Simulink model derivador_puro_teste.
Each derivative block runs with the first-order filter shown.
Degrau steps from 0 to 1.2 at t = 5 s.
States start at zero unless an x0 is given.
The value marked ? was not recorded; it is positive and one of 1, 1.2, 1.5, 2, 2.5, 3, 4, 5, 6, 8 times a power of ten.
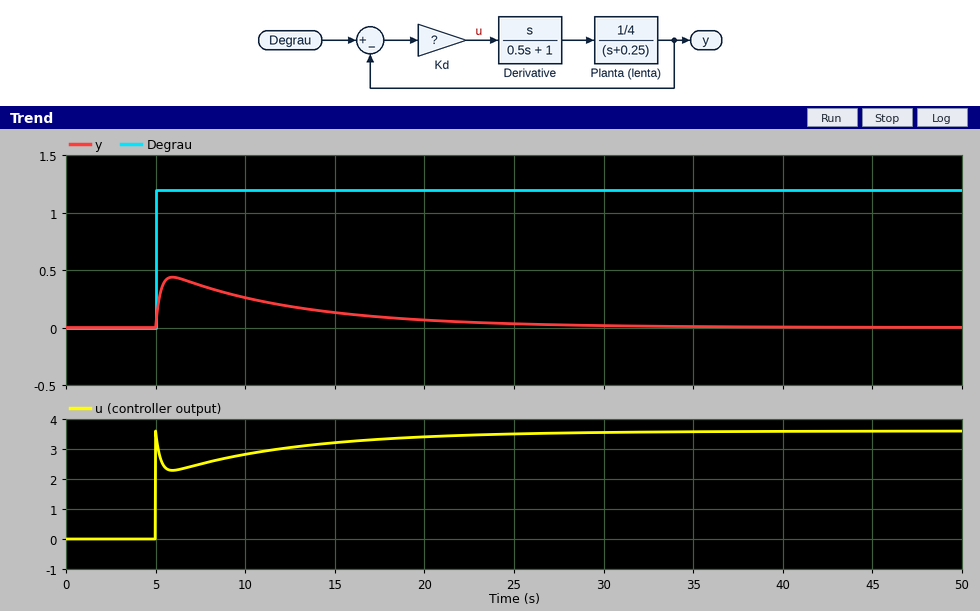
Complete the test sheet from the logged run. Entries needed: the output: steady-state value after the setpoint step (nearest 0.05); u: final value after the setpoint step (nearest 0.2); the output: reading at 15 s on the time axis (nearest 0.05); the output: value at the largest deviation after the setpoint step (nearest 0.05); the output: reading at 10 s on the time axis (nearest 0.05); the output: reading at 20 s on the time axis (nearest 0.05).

0.00
3.6
0.15
0.45
0.25
0.05
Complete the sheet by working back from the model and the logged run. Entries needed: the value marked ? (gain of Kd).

3
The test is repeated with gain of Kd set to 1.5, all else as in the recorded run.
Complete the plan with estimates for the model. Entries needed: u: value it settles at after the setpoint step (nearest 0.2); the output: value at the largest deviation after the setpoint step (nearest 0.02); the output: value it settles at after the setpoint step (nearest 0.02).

1.8
0.26
0.00
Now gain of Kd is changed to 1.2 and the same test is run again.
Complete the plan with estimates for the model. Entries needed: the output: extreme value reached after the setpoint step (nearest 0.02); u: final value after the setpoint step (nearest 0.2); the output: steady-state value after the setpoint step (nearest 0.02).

0.22
1.4
0.00
